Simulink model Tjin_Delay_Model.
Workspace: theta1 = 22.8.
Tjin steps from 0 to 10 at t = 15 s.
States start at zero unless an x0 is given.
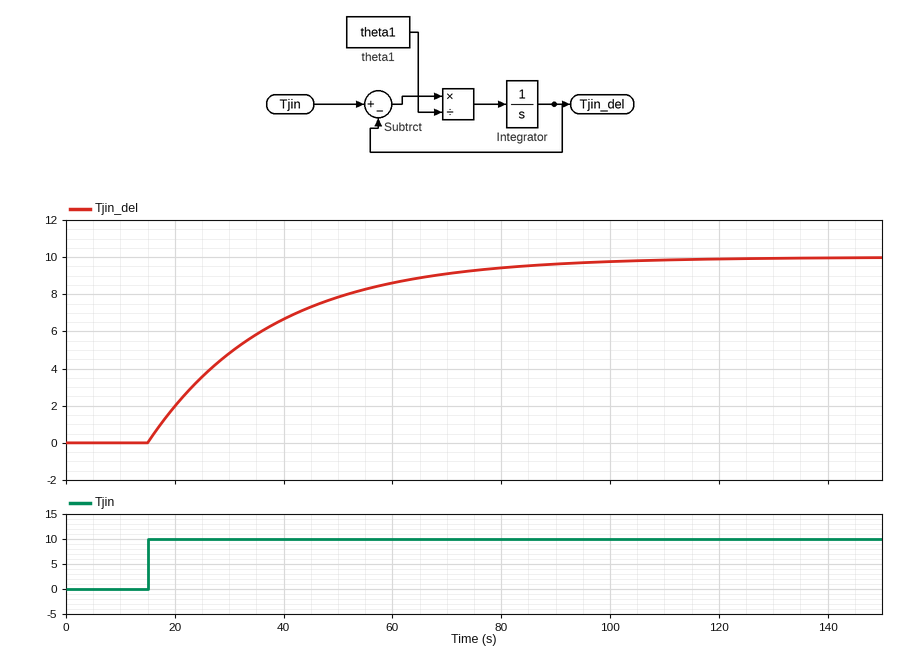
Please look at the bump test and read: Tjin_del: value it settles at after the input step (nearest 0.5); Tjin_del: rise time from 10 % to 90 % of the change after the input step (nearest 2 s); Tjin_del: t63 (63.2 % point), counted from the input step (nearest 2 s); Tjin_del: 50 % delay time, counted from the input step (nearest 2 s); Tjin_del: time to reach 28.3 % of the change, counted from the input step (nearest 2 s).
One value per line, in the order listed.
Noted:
10.0
50 s
22 s
16 s
8 s
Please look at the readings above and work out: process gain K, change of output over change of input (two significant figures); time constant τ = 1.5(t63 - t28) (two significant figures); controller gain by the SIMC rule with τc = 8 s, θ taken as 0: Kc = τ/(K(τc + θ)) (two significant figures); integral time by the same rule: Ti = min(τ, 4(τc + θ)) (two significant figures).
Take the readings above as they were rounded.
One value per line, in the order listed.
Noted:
1.0
21 s
2.6
21 s
